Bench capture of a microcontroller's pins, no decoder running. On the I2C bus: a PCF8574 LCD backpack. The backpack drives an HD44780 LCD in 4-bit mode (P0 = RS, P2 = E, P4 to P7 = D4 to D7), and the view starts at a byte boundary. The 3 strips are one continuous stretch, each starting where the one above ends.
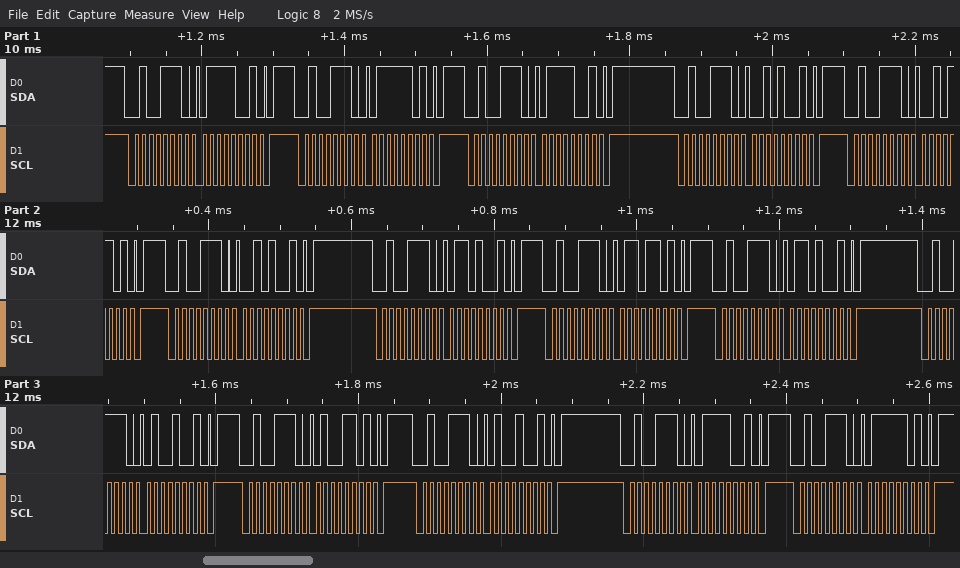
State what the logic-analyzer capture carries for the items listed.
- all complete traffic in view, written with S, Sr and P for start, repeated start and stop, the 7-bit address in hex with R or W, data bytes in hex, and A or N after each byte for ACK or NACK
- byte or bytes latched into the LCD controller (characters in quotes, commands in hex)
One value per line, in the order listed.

S 27W A 79 A P S 27W A 7D A P S 27W A 79 A P S 27W A 29 A P S 27W A 2D A P S 27W A 29 A P S 27W A 69 A P S 27W A 6D A P S 27W A 69 A P S 27W A 49 A P S 27W A 4D A P S 27W A 49 A P S 27W A 79 A P S 27W A 7D A P
'r' 'd'
